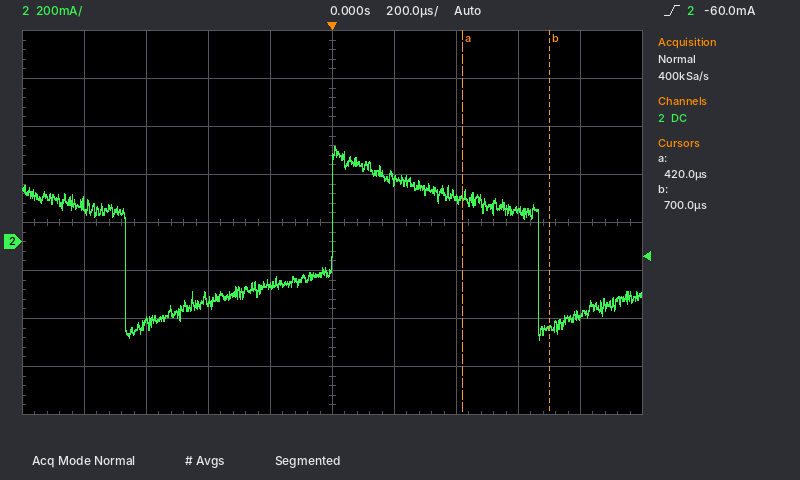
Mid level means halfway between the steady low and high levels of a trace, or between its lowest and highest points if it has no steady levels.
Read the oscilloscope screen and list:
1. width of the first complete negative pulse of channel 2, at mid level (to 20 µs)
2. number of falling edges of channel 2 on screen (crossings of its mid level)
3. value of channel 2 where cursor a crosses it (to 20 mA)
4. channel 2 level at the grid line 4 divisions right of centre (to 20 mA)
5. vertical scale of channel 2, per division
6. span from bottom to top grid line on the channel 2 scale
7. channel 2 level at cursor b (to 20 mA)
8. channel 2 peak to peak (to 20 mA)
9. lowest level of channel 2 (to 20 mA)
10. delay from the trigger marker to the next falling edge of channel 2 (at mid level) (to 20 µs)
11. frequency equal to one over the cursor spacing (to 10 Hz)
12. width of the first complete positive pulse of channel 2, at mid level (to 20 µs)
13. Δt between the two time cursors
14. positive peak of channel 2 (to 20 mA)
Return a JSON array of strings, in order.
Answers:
["660 µs", "2", "200 mA", "-300 mA", "200 mA", "1.6 A", "-360 mA", "800 mA", "-400 mA", "660 µs", "3.57 kHz", "660 µs", "280 µs", "400 mA"]
